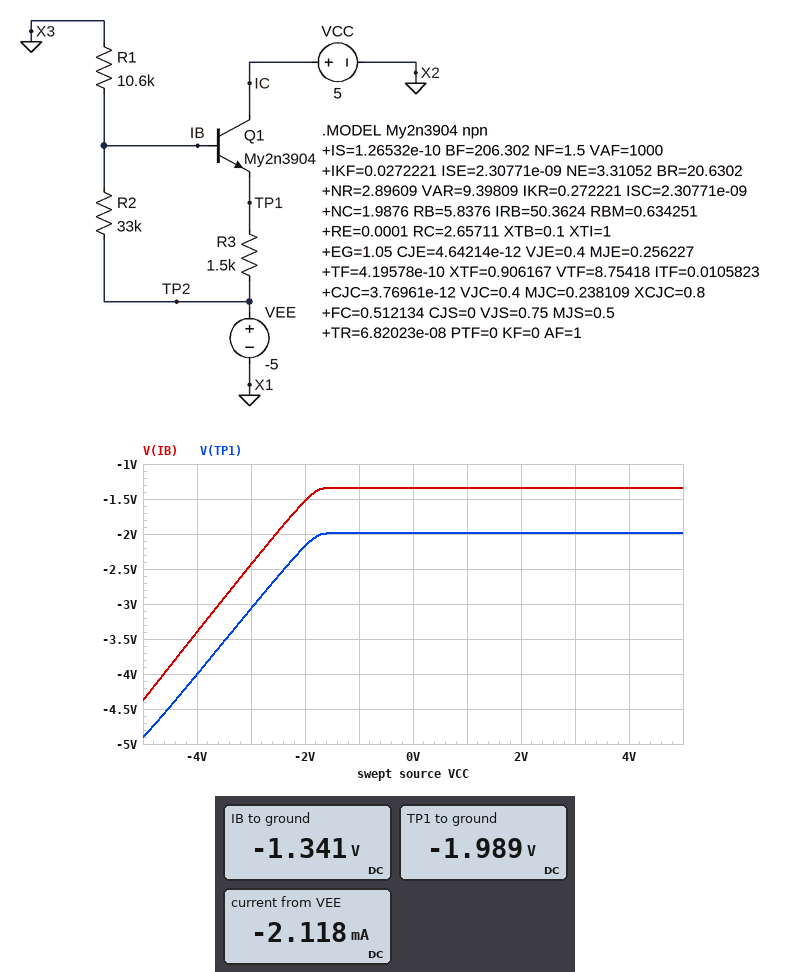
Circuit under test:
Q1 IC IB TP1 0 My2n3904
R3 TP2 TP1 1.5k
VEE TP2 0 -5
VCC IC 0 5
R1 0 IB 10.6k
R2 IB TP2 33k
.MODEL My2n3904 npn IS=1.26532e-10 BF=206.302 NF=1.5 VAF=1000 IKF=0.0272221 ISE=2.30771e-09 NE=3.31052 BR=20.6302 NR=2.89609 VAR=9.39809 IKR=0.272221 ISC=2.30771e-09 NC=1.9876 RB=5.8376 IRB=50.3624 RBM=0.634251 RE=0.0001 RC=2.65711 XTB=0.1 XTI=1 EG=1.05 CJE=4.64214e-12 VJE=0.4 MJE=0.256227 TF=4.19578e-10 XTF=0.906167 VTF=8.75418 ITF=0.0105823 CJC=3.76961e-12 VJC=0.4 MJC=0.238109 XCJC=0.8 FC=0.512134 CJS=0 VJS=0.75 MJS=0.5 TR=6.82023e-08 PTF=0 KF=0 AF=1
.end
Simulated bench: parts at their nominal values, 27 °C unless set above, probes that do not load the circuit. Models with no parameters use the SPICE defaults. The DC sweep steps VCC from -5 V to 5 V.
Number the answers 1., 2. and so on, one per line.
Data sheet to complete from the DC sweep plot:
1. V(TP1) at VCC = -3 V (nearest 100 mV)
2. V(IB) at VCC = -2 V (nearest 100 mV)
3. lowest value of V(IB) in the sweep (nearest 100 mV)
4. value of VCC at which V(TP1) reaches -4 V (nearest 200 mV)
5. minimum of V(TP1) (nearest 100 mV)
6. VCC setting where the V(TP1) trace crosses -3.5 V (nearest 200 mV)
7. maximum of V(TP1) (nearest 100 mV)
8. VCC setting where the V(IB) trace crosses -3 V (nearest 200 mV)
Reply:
1. -3.1 V
2. -1.5 V
3. -4.4 V
4. -4.0 V
5. -4.9 V
6. -3.4 V
7. -2.0 V
8. -3.6 V
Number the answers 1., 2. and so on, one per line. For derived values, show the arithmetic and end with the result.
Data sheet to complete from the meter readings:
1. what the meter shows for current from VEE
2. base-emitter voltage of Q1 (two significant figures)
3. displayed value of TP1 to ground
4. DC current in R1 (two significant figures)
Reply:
1. -2.118 mA
2. -1.341 V - (-1.989 V) = 650 mV
3. -1.989 V
4. (0 V - (-1.341 V)) / 10.6 kΩ = 130 µA
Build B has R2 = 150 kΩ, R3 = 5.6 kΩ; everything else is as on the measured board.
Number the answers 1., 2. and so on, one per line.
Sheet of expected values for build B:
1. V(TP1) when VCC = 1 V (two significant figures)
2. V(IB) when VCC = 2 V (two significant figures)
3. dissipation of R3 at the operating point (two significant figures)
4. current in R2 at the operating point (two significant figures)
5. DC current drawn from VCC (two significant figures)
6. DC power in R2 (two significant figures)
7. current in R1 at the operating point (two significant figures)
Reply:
1. -1.0 V
2. -390 mV
3. 2.9 mW
4. 31 µA
5. 710 µA
6. 140 µW
7. 37 µA
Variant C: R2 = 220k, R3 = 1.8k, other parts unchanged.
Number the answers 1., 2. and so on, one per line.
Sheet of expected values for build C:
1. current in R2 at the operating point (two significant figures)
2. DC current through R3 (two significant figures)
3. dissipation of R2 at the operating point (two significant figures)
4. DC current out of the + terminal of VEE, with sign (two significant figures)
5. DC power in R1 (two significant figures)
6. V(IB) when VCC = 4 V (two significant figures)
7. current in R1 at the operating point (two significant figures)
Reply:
1. 21 µA
2. 2.2 mA
3. 96 µW
4. -2.2 mA
5. 15 µW
6. -400 mV
7. 38 µA
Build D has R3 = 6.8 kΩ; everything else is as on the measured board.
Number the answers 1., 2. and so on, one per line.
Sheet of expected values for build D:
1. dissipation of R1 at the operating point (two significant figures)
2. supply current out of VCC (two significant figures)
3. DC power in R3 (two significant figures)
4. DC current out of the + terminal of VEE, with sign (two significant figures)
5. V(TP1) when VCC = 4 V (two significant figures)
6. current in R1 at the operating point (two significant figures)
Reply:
1. 150 µW
2. 460 µA
3. 1.5 mW
4. -580 µA
5. -1.8 V
6. 120 µA
